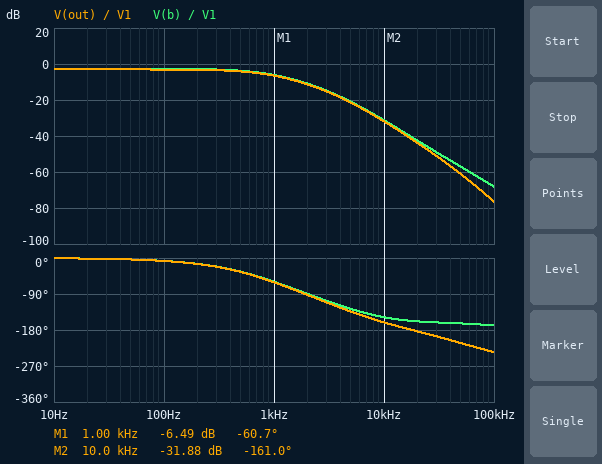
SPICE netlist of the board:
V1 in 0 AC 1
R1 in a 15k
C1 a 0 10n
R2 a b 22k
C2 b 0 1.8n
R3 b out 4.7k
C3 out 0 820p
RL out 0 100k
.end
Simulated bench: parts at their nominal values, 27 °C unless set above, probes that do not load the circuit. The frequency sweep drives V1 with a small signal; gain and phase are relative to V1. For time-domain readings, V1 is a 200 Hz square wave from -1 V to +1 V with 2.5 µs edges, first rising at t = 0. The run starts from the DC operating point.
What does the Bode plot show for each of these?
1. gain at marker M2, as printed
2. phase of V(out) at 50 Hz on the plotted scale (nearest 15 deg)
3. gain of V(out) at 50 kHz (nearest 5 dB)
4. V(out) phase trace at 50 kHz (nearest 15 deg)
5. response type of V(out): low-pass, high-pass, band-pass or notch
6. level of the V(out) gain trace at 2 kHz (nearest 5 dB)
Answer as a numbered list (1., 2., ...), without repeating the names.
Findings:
1. -31.88 dB
2. 0 deg
3. -60 dB
4. -210 deg
5. low-pass
6. -10 dB
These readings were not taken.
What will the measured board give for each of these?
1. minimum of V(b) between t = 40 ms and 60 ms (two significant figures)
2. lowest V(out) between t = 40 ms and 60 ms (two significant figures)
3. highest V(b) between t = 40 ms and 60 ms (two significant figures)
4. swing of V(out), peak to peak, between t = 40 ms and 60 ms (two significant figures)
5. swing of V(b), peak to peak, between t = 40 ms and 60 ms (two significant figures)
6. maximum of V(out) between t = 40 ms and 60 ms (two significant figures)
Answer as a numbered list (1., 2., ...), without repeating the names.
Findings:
1. -740 mV
2. -710 mV
3. 740 mV
4. 1.4 V
5. 1.5 V
6. 710 mV
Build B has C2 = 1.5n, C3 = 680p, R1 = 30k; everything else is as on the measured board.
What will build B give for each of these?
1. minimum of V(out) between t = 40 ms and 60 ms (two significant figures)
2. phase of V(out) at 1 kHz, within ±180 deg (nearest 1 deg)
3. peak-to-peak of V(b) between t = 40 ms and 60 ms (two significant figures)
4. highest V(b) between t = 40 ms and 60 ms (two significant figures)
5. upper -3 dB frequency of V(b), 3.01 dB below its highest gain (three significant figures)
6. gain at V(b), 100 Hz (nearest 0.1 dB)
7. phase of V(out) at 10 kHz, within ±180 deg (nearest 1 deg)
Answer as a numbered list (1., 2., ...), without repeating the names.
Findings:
1. -640 mV
2. -73 deg
3. 1.3 V
4. 670 mV
5. 554 Hz
6. -3.6 dB
7. -159 deg
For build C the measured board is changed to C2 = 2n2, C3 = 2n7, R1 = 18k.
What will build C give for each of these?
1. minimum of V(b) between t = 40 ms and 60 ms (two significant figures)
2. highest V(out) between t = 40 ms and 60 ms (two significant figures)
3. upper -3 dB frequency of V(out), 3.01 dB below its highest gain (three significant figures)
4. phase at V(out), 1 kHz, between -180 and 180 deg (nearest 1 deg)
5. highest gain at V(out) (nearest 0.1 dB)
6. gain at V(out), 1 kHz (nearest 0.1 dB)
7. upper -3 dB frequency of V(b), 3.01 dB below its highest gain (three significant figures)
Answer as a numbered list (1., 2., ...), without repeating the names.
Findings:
1. -720 mV
2. 690 mV
3. 629 Hz
4. -79 deg
5. -3.2 dB
6. -8.9 dB
7. 630 Hz
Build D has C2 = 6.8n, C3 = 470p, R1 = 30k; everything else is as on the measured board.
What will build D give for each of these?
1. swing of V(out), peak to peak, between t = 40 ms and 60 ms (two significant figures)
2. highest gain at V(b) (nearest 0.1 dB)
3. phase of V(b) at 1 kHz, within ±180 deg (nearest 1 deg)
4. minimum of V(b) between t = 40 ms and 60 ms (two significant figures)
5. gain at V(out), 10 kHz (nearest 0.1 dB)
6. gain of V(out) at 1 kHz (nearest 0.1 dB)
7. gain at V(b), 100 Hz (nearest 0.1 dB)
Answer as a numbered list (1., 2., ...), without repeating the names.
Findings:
1. 1.3 V
2. -3.5 dB
3. -95 deg
4. -660 mV
5. -46.2 dB
6. -13.8 dB
7. -3.8 dB
